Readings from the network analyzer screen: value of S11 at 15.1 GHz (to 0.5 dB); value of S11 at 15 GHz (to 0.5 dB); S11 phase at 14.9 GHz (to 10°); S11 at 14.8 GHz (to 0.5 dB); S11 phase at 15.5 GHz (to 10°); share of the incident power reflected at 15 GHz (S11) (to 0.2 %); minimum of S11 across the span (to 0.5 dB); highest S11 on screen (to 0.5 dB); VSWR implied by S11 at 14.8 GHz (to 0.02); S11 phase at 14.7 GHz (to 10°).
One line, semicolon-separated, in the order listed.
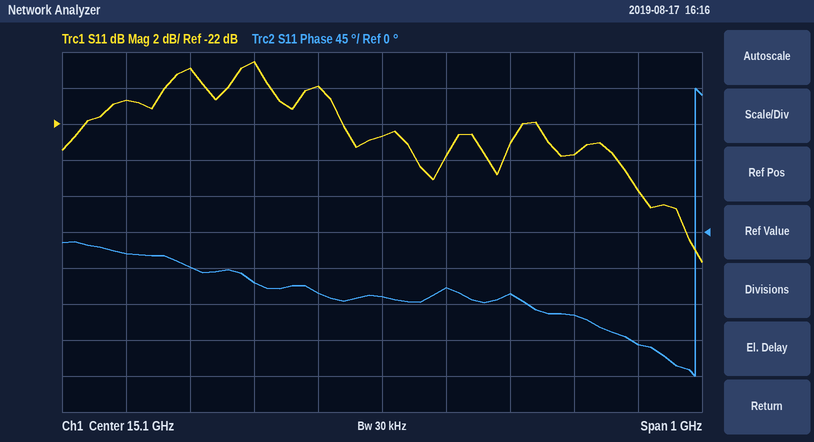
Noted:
-22.5 dB; -20.0 dB; -60°; -19.0 dB; -140°; 1.0 %; -29.5 dB; -18.5 dB; 1.26; -30°
